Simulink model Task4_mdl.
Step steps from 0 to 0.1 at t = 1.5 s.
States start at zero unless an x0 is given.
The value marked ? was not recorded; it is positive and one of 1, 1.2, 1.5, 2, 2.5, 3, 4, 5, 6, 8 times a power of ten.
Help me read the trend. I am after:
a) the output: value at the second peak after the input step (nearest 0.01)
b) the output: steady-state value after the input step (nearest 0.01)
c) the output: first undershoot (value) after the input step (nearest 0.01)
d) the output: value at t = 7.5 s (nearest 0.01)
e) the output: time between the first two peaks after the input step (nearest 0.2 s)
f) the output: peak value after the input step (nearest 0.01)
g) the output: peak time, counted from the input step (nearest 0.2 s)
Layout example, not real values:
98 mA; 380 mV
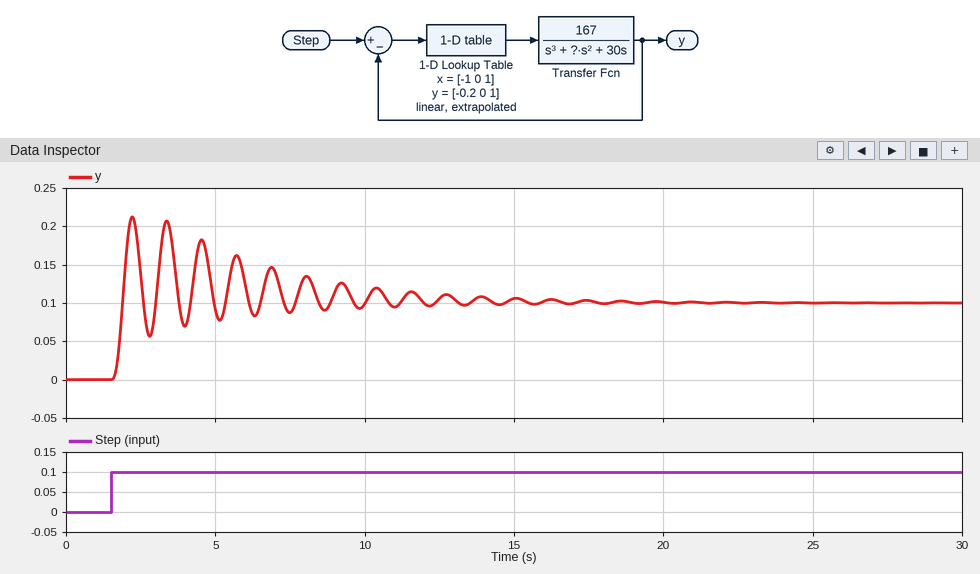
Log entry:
0.21; 0.10; 0.06; 0.09; 1.2 s; 0.21; 0.8 s
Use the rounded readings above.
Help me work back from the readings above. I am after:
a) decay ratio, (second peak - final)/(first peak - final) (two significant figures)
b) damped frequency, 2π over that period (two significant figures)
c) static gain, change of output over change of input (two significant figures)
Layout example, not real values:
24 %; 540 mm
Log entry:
1.0; 5.2 rad/s; 1.0
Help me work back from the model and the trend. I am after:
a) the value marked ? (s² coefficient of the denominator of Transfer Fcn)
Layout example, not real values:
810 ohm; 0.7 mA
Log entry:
2.5
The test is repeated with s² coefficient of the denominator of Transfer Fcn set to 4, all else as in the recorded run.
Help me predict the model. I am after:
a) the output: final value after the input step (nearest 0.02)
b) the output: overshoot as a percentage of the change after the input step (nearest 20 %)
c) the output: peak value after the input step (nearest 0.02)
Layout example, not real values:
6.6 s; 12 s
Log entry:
0.10; 100 %; 0.20
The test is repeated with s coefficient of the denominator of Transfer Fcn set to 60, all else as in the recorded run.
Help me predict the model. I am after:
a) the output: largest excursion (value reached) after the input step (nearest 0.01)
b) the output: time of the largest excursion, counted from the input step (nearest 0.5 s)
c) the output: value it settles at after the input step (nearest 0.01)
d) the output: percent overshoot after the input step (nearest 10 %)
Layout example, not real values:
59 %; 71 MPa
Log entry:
0.13; 1.5 s; 0.10; 30 %
